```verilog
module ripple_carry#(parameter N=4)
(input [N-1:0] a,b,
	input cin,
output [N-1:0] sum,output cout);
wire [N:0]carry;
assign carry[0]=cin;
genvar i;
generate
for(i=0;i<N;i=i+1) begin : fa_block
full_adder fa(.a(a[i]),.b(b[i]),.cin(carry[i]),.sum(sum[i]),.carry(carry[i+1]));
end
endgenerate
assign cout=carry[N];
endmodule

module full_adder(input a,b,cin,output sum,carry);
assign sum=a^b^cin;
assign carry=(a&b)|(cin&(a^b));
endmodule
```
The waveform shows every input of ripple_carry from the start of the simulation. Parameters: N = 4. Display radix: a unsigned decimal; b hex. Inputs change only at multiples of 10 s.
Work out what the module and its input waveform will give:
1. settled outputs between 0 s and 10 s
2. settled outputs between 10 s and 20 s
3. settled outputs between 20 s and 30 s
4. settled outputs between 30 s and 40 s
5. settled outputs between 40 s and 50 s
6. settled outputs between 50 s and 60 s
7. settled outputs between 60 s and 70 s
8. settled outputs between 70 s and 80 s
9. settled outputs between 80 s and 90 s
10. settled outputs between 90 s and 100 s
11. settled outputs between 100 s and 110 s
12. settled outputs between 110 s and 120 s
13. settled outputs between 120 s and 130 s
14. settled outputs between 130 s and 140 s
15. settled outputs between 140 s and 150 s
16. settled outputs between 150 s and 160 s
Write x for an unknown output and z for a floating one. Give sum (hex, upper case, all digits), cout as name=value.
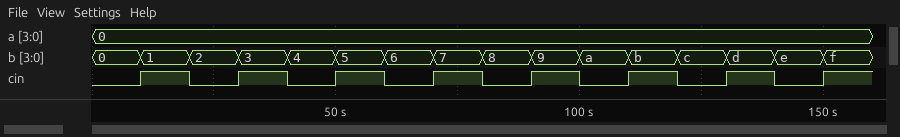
sum=0, cout=0
sum=2, cout=0
sum=2, cout=0
sum=4, cout=0
sum=4, cout=0
sum=6, cout=0
sum=6, cout=0
sum=8, cout=0
sum=8, cout=0
sum=A, cout=0
sum=A, cout=0
sum=C, cout=0
sum=C, cout=0
sum=E, cout=0
sum=E, cout=0
sum=0, cout=1
